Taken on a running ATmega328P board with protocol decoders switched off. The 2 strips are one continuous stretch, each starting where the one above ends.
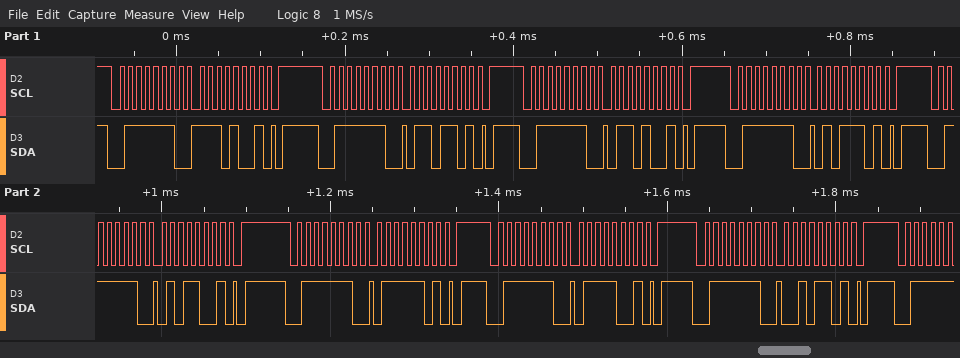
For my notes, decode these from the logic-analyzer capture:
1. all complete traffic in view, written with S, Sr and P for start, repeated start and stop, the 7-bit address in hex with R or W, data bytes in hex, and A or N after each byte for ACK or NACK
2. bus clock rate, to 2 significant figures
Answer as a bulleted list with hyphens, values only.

- S 3FW A E9 A P S 3FW A 6D A P S 3FW A 69 A P S 3FW A 5D A P S 3FW A 59 A P S 3FW A 7D A P S 3FW A 79 A P S 3FW A 2D A P
- 100 kHz
